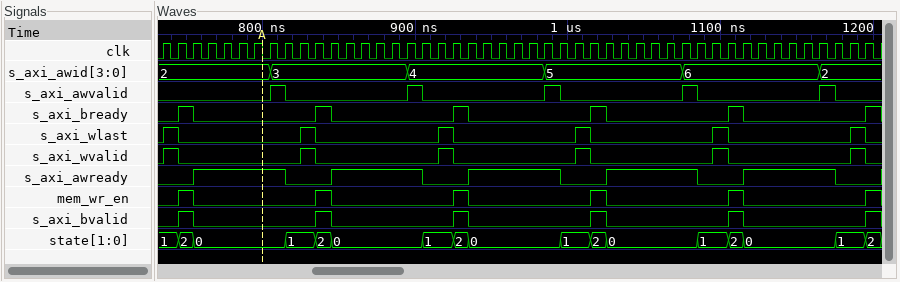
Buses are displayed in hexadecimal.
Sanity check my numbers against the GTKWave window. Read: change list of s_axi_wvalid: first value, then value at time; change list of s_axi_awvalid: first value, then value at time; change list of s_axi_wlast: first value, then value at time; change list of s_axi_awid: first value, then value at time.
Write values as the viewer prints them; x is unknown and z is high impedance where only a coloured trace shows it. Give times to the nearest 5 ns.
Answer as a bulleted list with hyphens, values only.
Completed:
- 0, 1 at 735 ns, 0 at 745 ns, 1 at 825 ns, 0 at 835 ns, 1 at 915 ns, 0 at 925 ns, 1 at 1005 ns, 0 at 1015 ns, 1 at 1095 ns, 0 at 1105 ns, 1 at 1185 ns, 0 at 1195 ns
- 0, 1 at 805 ns, 0 at 815 ns, 1 at 895 ns, 0 at 905 ns, 1 at 985 ns, 0 at 995 ns, 1 at 1075 ns, 0 at 1085 ns, 1 at 1165 ns, 0 at 1175 ns
- 0, 1 at 735 ns, 0 at 745 ns, 1 at 825 ns, 0 at 835 ns, 1 at 915 ns, 0 at 925 ns, 1 at 1005 ns, 0 at 1015 ns, 1 at 1095 ns, 0 at 1105 ns, 1 at 1185 ns, 0 at 1195 ns
- 2, 3 at 805 ns, 4 at 895 ns, 5 at 985 ns, 6 at 1075 ns, 2 at 1165 ns
